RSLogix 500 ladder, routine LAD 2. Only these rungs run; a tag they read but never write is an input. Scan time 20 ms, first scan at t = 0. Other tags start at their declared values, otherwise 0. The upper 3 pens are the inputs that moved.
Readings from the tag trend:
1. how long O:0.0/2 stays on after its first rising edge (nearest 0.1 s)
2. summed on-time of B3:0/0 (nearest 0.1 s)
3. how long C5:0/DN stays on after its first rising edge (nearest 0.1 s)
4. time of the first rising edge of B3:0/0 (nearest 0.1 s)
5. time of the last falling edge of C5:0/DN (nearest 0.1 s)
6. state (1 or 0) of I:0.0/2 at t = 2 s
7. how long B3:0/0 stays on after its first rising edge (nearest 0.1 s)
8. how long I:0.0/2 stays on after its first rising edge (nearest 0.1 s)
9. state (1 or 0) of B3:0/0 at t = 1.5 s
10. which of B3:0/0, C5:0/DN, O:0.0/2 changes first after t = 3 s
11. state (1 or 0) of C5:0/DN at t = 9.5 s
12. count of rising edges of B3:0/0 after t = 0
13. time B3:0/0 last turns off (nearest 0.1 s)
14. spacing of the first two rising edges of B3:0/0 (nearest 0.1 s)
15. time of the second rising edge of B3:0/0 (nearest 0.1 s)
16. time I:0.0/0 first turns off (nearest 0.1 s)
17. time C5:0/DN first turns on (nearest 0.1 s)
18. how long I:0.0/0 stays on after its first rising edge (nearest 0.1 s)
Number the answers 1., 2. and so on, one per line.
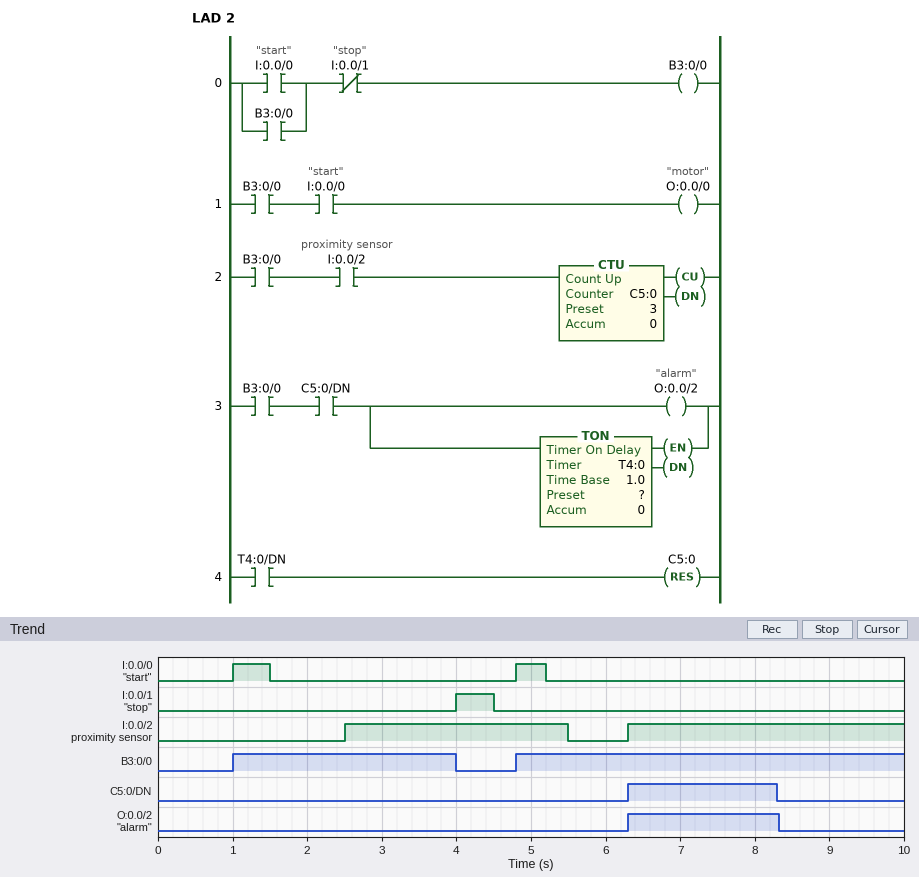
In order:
1. 2.0 s
2. 8.2 s
3. 2.0 s
4. 1.0 s
5. 8.3 s
6. 0
7. 3.0 s
8. 3.0 s
9. 1
10. B3:0/0
11. 0
12. 2
13. 4.0 s
14. 3.8 s
15. 4.8 s
16. 1.5 s
17. 6.3 s
18. 0.5 s
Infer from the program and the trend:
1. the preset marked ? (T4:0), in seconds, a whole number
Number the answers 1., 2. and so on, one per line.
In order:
1. 2 s
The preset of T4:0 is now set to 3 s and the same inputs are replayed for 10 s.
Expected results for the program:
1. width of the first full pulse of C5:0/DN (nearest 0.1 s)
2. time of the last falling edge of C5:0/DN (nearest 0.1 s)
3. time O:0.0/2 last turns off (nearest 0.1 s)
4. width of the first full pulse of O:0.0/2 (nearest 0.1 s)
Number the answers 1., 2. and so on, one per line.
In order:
1. 3.0 s
2. 9.3 s
3. 9.3 s
4. 3.0 s
